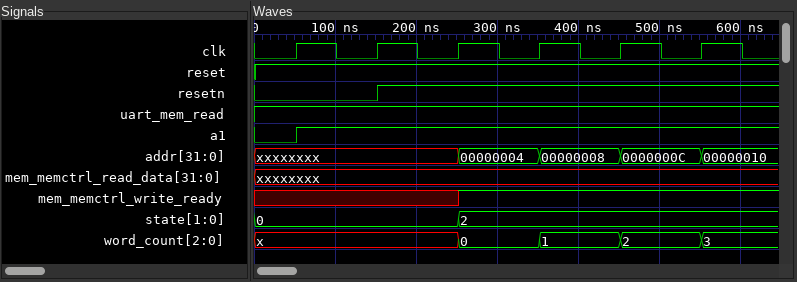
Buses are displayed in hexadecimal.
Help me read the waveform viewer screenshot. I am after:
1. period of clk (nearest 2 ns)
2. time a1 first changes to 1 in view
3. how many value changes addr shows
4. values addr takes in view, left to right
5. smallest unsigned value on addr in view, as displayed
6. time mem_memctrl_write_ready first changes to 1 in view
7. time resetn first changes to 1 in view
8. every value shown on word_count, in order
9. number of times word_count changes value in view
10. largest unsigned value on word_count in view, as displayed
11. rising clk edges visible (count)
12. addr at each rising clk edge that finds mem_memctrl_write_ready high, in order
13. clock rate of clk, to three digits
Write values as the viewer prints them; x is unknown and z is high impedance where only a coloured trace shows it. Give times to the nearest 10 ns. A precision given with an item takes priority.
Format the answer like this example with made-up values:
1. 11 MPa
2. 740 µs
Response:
1. 100 ns
2. 50 ns
3. 4
4. xxxxxxxx, 00000004, 00000008, 0000000C, 00000010
5. 00000004
6. 250 ns
7. 150 ns
8. x, 0, 1, 2, 3
9. 4
10. 3
11. 6
12. 00000004, 00000008, 0000000C
13. 10.0 MHz
